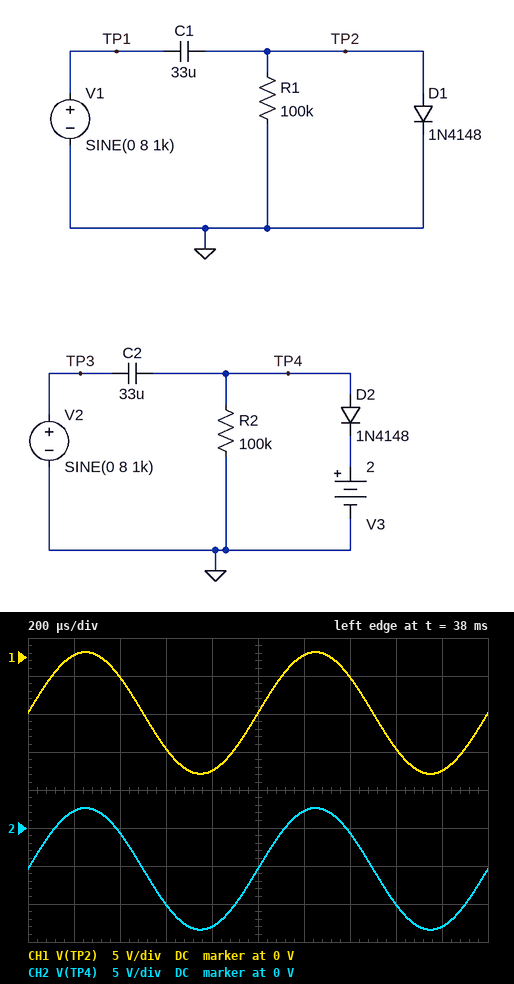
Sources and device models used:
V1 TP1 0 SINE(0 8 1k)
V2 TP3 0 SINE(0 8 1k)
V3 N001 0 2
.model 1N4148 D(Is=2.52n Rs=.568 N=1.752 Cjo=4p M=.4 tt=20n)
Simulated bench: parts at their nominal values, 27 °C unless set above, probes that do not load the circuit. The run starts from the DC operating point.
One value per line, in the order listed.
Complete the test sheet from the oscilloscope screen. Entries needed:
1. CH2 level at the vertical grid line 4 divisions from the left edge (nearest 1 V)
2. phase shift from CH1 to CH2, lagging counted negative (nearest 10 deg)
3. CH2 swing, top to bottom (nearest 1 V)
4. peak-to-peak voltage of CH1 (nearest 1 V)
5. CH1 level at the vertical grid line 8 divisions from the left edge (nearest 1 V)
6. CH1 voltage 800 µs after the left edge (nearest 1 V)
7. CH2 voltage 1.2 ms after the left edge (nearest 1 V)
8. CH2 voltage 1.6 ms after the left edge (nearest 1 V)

-13 V
0 deg
16 V
16 V
-12 V
-15 V
2 V
-10 V
